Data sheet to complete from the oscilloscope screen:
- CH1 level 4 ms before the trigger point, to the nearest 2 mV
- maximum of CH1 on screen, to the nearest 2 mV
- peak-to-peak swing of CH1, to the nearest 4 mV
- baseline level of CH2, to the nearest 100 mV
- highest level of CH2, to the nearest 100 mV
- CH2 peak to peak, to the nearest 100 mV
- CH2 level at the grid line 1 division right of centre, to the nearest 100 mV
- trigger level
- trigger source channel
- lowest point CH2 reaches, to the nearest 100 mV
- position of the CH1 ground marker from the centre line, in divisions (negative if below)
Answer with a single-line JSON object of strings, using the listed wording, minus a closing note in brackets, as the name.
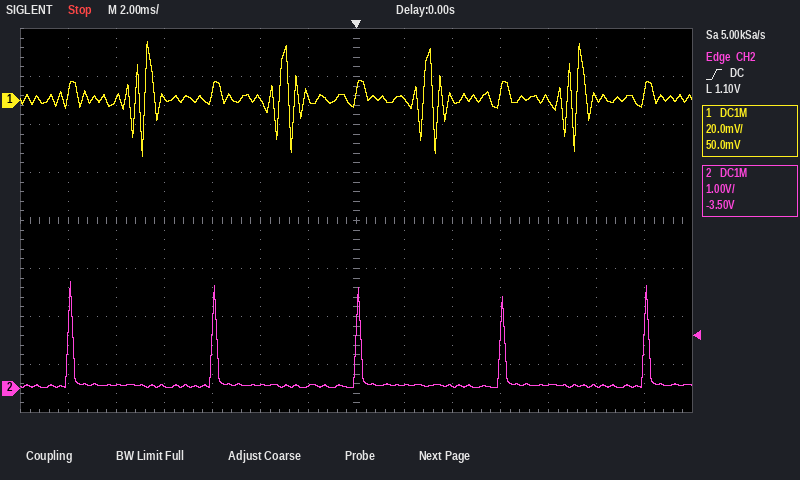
{"CH1 level 4 ms before the trigger point, to the nearest 2 mV": "0 mV", "maximum of CH1 on screen, to the nearest 2 mV": "24 mV", "peak-to-peak swing of CH1, to the nearest 4 mV": "48 mV", "baseline level of CH2, to the nearest 100 mV": "100 mV", "highest level of CH2, to the nearest 100 mV": "2.2 V", "CH2 peak to peak, to the nearest 100 mV": "2.2 V", "CH2 level at the grid line 1 division right of centre, to the nearest 100 mV": "100 mV", "trigger level": "1.10 V", "trigger source channel": "CH2", "lowest point CH2 reaches, to the nearest 100 mV": "0.0 V", "position of the CH1 ground marker from the centre line, in divisions": "+2.5 div"}
